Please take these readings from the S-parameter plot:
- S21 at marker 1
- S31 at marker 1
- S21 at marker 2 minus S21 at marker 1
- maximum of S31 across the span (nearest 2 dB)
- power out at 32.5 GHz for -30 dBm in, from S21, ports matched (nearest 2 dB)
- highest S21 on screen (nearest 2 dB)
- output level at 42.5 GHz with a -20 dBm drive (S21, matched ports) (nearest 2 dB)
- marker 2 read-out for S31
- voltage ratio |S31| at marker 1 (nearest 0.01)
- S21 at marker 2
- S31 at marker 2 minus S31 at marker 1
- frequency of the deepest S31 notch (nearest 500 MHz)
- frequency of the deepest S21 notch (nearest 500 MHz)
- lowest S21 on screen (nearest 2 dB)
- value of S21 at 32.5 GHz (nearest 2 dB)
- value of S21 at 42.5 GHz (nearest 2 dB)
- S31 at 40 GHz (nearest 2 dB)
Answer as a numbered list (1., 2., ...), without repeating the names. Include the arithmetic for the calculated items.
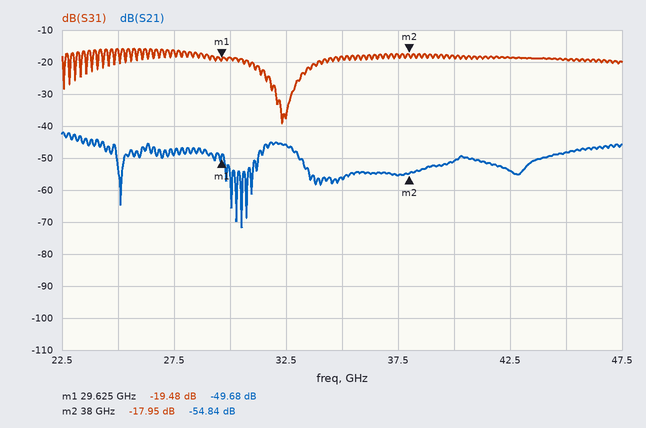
1. -49.68 dB
2. -19.48 dB
3. -54.84 − (-49.68) = -5.16 dB
4. -16 dB
5. -30 dBm + (-46 dB) = -76 dBm
6. -42 dB
7. -20 dBm + (-54 dB) = -74 dBm
8. -17.95 dB
9. 10^(-19.48/20) ≈ 0.11
10. -54.84 dB
11. -17.95 − (-19.48) = 1.53 dB
12. 32.5 GHz
13. 30.5 GHz
14. -72 dB
15. -46 dB
16. -54 dB
17. -18 dB
